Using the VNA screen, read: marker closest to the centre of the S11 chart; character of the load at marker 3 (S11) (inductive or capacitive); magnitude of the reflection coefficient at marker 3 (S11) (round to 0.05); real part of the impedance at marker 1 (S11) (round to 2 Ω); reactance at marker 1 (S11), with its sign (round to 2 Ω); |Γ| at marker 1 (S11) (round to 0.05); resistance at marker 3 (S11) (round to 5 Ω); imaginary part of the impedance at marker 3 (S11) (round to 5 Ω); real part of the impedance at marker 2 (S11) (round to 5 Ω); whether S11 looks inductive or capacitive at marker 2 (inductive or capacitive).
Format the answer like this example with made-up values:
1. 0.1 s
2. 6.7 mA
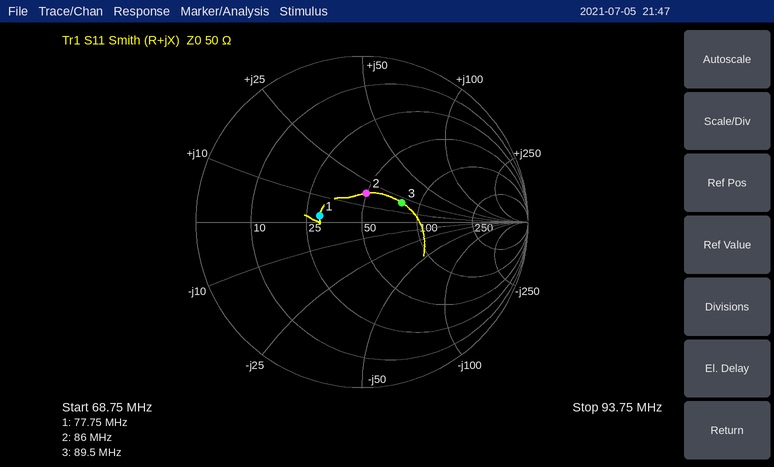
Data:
1. marker 2
2. inductive
3. 0.25
4. 30 Ω
5. +2 Ω
6. 0.25
7. 80 Ω
8. +20 Ω
9. 50 Ω
10. inductive
